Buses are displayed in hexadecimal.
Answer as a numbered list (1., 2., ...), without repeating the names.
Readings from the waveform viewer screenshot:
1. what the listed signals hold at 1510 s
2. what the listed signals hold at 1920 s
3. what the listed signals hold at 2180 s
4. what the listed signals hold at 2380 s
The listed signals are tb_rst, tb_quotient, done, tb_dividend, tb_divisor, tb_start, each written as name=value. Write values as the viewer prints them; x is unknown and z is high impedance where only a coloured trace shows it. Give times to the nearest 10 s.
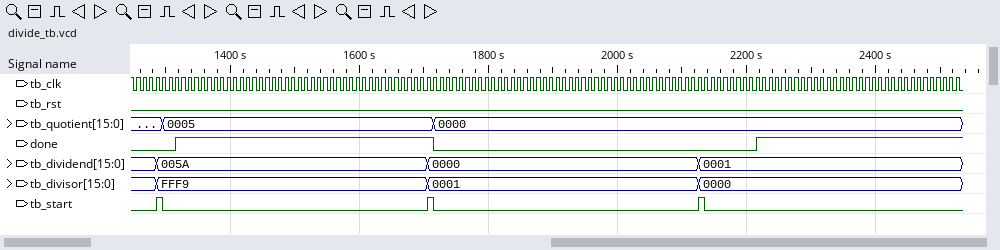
1. tb_rst=0, tb_quotient=0005, done=1, tb_dividend=005A, tb_divisor=FFF9, tb_start=0
2. tb_rst=0, tb_quotient=0000, done=0, tb_dividend=0000, tb_divisor=0001, tb_start=0
3. tb_rst=0, tb_quotient=0000, done=0, tb_dividend=0001, tb_divisor=0000, tb_start=0
4. tb_rst=0, tb_quotient=0000, done=1, tb_dividend=0001, tb_divisor=0000, tb_start=0
